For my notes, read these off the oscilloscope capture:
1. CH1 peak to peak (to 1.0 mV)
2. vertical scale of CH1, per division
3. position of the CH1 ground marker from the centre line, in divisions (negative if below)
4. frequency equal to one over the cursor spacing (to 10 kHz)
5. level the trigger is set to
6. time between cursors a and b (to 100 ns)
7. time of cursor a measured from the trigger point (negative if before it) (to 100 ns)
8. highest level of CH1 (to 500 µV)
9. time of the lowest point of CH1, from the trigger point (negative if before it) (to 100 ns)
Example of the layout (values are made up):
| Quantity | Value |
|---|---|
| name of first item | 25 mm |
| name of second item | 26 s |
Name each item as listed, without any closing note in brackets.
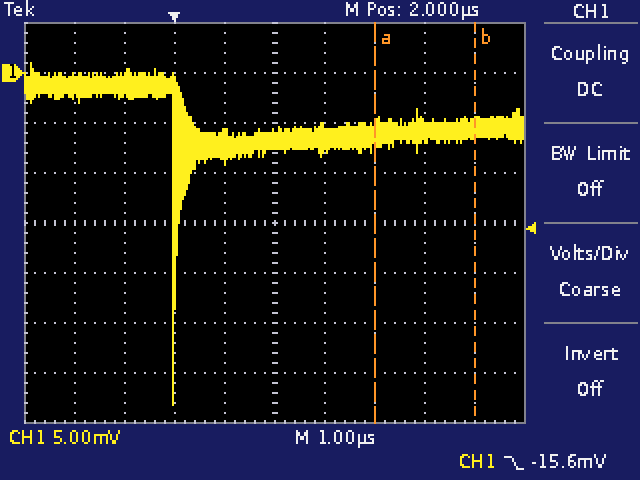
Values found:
| Quantity | Value |
|---|---|
| CH1 peak to peak | 34.0 mV |
| vertical scale of CH1, per division | 5 mV |
| position of the CH1 ground marker from the centre line, in divisions | +3.0 div |
| frequency equal to one over the cursor spacing | 500 kHz |
| level the trigger is set to | -15.6 mV |
| time between cursors a and b | 2.0 µs |
| time of cursor a measured from the trigger point (negative if before it) | +4.0 µs |
| highest level of CH1 | 1.0 mV |
| time of the lowest point of CH1, from the trigger point (negative if before it) | 0.0 µs |
